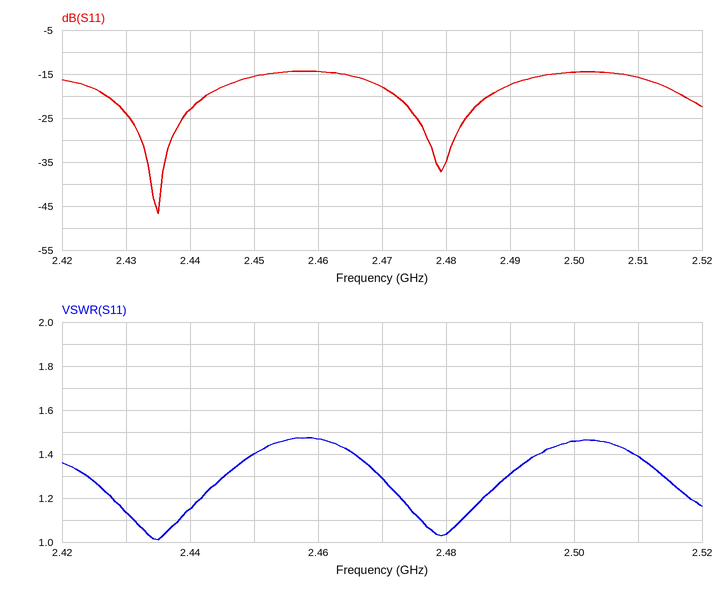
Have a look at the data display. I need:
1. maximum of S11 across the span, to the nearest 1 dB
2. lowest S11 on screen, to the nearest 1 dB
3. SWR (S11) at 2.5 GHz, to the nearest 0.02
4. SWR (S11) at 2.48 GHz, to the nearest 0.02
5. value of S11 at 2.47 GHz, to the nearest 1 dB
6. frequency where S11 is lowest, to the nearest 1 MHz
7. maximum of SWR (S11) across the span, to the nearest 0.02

-14 dB
-47 dB
1.46
1.04
-18 dB
2.435 GHz
1.48
